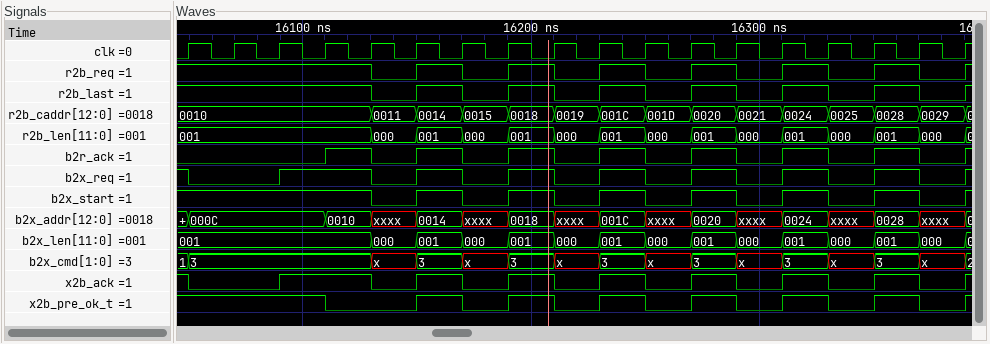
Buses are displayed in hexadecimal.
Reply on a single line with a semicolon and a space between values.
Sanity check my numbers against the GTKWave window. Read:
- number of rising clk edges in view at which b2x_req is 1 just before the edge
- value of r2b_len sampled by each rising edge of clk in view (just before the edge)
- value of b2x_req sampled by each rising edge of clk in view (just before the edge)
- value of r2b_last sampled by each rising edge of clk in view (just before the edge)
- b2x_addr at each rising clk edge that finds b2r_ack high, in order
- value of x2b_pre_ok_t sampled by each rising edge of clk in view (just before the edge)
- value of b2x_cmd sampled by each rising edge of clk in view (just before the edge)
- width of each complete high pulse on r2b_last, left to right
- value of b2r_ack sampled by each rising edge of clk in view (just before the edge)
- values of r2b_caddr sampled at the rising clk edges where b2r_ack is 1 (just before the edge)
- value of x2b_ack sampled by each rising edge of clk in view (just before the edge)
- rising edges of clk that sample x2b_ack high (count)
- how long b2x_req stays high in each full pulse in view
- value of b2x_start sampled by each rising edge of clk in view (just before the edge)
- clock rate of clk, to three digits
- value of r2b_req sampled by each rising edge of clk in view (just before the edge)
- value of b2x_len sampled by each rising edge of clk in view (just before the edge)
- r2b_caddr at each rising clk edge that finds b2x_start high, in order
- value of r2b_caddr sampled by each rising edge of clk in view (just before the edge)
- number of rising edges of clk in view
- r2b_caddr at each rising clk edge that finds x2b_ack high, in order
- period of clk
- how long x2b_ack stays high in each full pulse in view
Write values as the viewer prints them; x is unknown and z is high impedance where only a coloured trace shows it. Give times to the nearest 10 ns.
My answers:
9; 001, 001, 001, 001, 001, 000, 001, 000, 001, 000, 001, 000, 001, 000, 001, 000, 001, 000; 1 0 0 1 1 0 1 0 1 0 1 0 1 0 1 0 1 0; 1 1 1 1 1 0 1 0 1 0 1 0 1 0 1 0 1 0; 0010, 0014, 0018, 001C, 0020, 0024, 0028; 1 1 1 1 0 0 1 0 1 0 1 0 1 0 1 0 1 0; 1, 3, 3, 3, 3, x, 3, x, 3, x, 3, x, 3, x, 3, x, 3, x; 20 ns, 20 ns, 20 ns, 20 ns, 20 ns, 20 ns; 0 0 0 0 1 0 1 0 1 0 1 0 1 0 1 0 1 0; 0010, 0014, 0018, 001C, 0020, 0024, 0028; 1 0 0 1 1 0 1 0 1 0 1 0 1 0 1 0 1 0; 9; 40 ns, 20 ns, 20 ns, 20 ns, 20 ns, 20 ns, 20 ns; 1 1 1 1 1 0 1 0 1 0 1 0 1 0 1 0 1 0; 50.0 MHz; 1 1 1 1 1 0 1 0 1 0 1 0 1 0 1 0 1 0; 001, 001, 001, 001, 001, 000, 001, 000, 001, 000, 001, 000, 001, 000, 001, 000, 001, 000; 0010, 0010, 0010, 0010, 0010, 0014, 0018, 001C, 0020, 0024, 0028; 0010, 0010, 0010, 0010, 0010, 0011, 0014, 0015, 0018, 0019, 001C, 001D, 0020, 0021, 0024, 0025, 0028, 0029; 18; 0010, 0010, 0010, 0014, 0018, 001C, 0020, 0024, 0028; 20 ns; 40 ns, 20 ns, 20 ns, 20 ns, 20 ns, 20 ns, 20 ns
